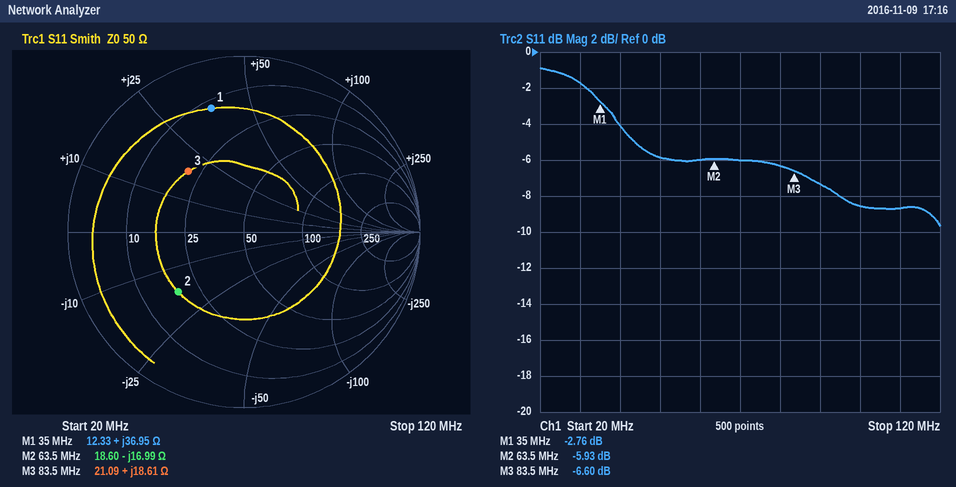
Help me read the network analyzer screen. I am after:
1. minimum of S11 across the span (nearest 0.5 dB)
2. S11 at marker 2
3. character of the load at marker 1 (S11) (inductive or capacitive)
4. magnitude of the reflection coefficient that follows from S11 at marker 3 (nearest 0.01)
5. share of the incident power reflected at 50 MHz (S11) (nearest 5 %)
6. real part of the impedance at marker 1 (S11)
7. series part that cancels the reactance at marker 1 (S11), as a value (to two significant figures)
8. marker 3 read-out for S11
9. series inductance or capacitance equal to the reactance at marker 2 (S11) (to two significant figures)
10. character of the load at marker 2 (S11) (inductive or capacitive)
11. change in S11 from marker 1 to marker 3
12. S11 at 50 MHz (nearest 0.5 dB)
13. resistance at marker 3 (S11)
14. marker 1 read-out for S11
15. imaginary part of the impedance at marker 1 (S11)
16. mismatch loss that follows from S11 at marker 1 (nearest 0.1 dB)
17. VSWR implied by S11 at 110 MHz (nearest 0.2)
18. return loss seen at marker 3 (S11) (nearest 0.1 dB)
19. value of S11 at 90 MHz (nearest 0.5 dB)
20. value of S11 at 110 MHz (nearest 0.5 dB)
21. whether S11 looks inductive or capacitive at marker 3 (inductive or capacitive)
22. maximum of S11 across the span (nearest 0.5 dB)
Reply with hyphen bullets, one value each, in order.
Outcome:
- -9.5 dB
- -5.93 dB
- inductive
- 0.47
- 25 %
- 12.33 Ω
- 120 pF
- -6.60 dB
- 150 pF
- capacitive
- -3.84 dB
- -6.0 dB
- 21.09 Ω
- -2.76 dB
- +36.95 Ω
- 3.3 dB
- 2.2
- 6.6 dB
- -7.5 dB
- -8.5 dB
- inductive
- -1.0 dB
